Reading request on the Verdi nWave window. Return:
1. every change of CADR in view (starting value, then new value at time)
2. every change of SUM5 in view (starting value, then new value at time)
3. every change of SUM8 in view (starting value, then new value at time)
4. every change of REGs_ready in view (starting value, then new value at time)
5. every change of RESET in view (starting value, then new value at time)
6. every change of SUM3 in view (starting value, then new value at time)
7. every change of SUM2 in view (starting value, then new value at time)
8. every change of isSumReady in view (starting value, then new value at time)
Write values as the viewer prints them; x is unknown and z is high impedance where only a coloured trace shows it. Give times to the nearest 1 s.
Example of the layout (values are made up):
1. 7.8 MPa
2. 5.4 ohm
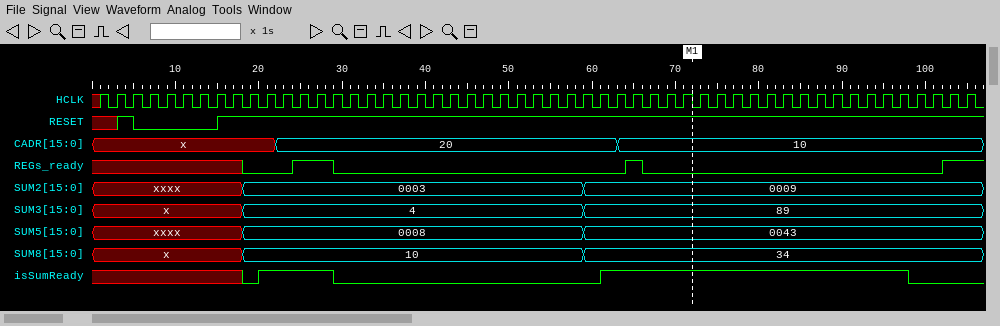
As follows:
1. x, 20 at 22 s, 10 at 63 s
2. xxxx, 0008 at 18 s, 0043 at 59 s
3. x, 10 at 18 s, 34 at 59 s
4. x, 0 at 18 s, 1 at 24 s, 0 at 29 s, 1 at 64 s, 0 at 66 s, 1 at 102 s
5. x, 1 at 3 s, 0 at 5 s, 1 at 15 s
6. x, 4 at 18 s, 89 at 59 s
7. xxxx, 0003 at 18 s, 0009 at 59 s
8. x, 0 at 18 s, 1 at 20 s, 0 at 29 s, 1 at 61 s, 0 at 98 s
